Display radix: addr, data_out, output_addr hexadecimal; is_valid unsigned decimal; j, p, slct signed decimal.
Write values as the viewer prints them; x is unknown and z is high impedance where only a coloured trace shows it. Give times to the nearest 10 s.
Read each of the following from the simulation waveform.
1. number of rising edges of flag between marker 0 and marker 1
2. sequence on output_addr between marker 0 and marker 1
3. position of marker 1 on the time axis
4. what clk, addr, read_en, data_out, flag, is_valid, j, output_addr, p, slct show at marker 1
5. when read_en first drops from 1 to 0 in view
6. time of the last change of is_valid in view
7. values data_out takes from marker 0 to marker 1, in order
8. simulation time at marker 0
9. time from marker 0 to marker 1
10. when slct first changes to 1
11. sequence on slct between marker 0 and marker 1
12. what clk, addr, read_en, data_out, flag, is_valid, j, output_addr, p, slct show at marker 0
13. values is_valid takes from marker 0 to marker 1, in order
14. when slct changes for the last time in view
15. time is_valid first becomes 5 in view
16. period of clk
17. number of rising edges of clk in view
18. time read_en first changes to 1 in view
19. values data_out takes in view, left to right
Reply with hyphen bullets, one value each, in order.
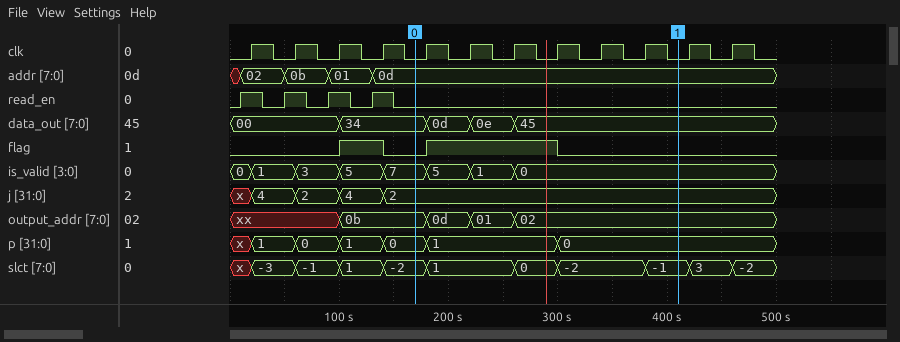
- 1
- 0b, 0d, 01, 02
- 410 s
- clk=0, addr=0d, read_en=0, data_out=45, flag=0, is_valid=0, j=2, output_addr=02, p=0, slct=-1
- 30 s
- 260 s
- 34, 0d, 0e, 45
- 170 s
- 240 s
- 100 s
- -2, 1, 0, -2, -1
- clk=0, addr=0d, read_en=0, data_out=34, flag=0, is_valid=7, j=2, output_addr=0b, p=0, slct=-2
- 7, 5, 1, 0
- 460 s
- 100 s
- 40 s
- 12
- 10 s
- 00, 34, 0d, 0e, 45
